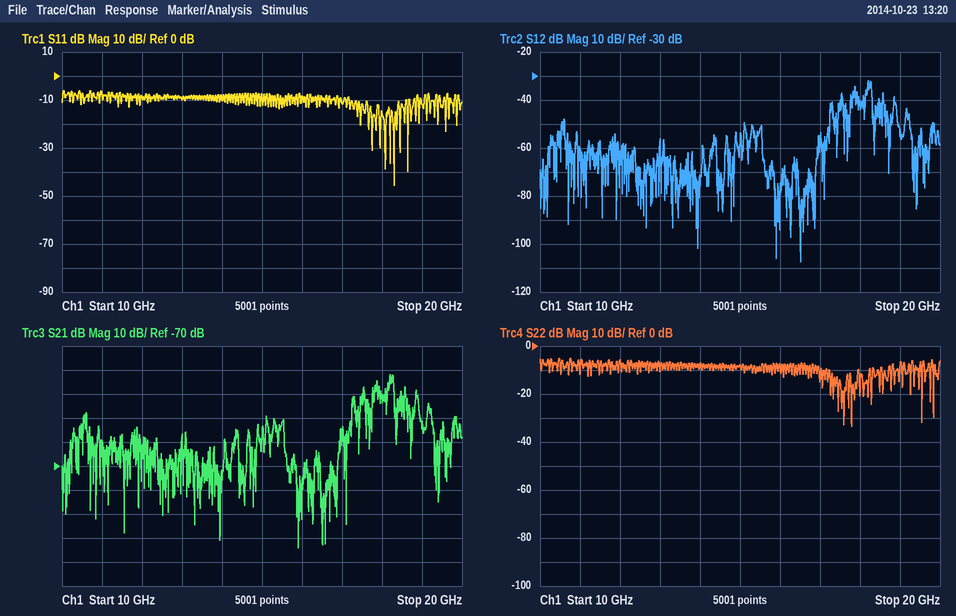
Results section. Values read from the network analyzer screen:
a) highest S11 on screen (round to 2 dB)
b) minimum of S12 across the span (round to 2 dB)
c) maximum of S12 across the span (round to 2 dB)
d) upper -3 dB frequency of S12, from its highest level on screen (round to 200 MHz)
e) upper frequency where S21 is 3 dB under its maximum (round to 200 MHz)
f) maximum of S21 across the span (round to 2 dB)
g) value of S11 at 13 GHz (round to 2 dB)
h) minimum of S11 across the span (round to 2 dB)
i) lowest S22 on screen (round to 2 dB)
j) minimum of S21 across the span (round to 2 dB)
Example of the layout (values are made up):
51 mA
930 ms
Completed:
-6 dB
-108 dB
-32 dB
18.2 GHz
18.2 GHz
-32 dB
-10 dB
-46 dB
-34 dB
-104 dB
